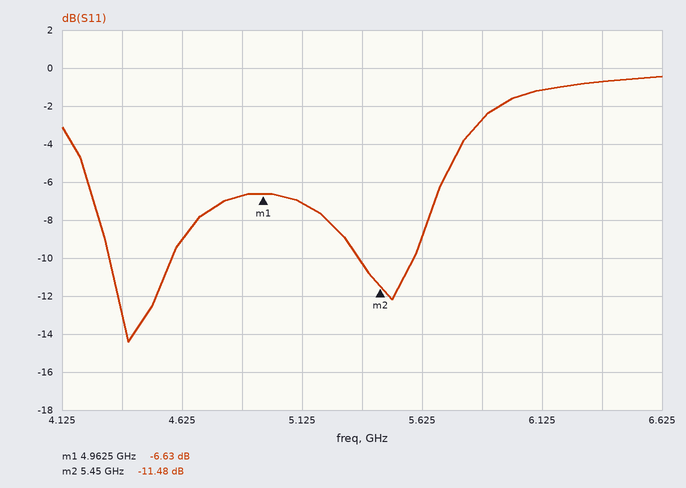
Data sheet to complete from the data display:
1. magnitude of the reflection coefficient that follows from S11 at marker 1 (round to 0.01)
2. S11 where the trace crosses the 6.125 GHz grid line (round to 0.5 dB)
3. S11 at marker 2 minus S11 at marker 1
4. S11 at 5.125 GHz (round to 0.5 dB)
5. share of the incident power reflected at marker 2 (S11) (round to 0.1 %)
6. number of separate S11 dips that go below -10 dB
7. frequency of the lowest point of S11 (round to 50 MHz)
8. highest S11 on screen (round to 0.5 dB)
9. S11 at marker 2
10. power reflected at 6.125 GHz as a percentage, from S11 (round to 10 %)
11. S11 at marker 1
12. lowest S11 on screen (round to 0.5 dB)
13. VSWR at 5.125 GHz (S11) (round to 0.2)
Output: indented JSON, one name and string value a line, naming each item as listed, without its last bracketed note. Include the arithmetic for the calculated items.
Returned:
{
  "magnitude of the reflection coefficient that follows from S11 at marker 1": "10^(-6.63/20) ≈ 0.47",
  "S11 where the trace crosses the 6.125 GHz grid line": "-1.0 dB",
  "S11 at marker 2 minus S11 at marker 1": "-11.48 − (-6.63) = -4.85 dB",
  "S11 at 5.125 GHz": "-7.0 dB",
  "share of the incident power reflected at marker 2 (S11)": "10^(-11.48/10) ≈ 7.1 %",
  "number of separate S11 dips that go below -10 dB": "2",
  "frequency of the lowest point of S11": "4.40 GHz",
  "highest S11 on screen": "-0.5 dB",
  "S11 at marker 2": "-11.48 dB",
  "power reflected at 6.125 GHz as a percentage, from S11": "10^(-1/10) ≈ 79.4 %, so 80 % to the nearest 10 %",
  "S11 at marker 1": "-6.63 dB",
  "lowest S11 on screen": "-14.5 dB",
  "VSWR at 5.125 GHz (S11)": "|Γ| = 10^(-7/20) = 0.4467; VSWR = (1 + 0.4467)/(1 − 0.4467) ≈ 2.6"
}
